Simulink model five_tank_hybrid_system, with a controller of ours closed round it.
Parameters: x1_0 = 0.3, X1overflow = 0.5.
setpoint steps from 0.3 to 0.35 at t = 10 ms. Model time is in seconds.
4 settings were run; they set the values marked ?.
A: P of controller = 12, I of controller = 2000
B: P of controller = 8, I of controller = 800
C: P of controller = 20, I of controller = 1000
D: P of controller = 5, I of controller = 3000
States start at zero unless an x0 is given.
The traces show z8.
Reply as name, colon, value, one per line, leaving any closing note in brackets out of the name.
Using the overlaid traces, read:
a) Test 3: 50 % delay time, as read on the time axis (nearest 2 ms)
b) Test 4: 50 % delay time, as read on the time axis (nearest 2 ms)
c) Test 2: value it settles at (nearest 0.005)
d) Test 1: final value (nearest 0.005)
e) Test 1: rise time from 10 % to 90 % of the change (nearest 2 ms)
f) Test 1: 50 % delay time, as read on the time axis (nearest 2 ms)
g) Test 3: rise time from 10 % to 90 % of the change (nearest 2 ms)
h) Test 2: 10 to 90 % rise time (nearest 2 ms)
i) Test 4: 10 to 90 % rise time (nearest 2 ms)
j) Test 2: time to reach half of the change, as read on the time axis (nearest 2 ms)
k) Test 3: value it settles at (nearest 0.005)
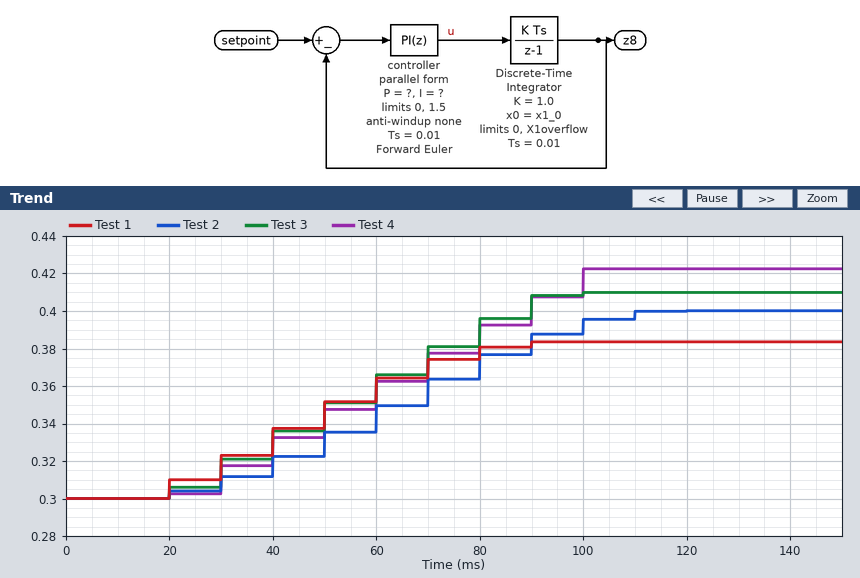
Test 3: 50 % delay time, as read on the time axis: 60 ms
Test 4: 50 % delay time, as read on the time axis: 60 ms
Test 2: value it settles at: 0.400
Test 1: final value: 0.385
Test 1: rise time from 10 % to 90 % of the change: 60 ms
Test 1: 50 % delay time, as read on the time axis: 50 ms
Test 3: rise time from 10 % to 90 % of the change: 60 ms
Test 2: 10 to 90 % rise time: 70 ms
Test 4: 10 to 90 % rise time: 70 ms
Test 2: time to reach half of the change, as read on the time axis: 70 ms
Test 3: value it settles at: 0.410
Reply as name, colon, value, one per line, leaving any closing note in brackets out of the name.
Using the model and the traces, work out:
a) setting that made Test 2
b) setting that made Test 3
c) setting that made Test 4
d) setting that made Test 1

setting that made Test 2: B
setting that made Test 3: A
setting that made Test 4: D
setting that made Test 1: C
